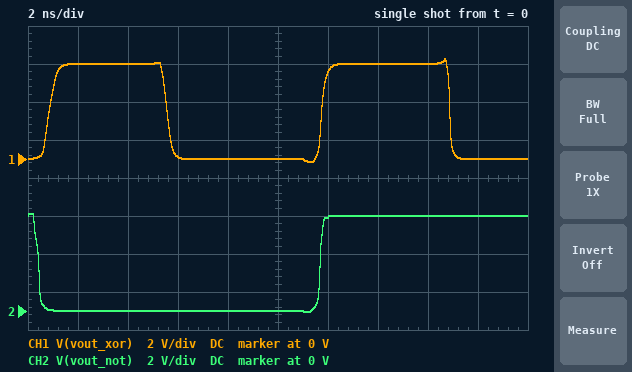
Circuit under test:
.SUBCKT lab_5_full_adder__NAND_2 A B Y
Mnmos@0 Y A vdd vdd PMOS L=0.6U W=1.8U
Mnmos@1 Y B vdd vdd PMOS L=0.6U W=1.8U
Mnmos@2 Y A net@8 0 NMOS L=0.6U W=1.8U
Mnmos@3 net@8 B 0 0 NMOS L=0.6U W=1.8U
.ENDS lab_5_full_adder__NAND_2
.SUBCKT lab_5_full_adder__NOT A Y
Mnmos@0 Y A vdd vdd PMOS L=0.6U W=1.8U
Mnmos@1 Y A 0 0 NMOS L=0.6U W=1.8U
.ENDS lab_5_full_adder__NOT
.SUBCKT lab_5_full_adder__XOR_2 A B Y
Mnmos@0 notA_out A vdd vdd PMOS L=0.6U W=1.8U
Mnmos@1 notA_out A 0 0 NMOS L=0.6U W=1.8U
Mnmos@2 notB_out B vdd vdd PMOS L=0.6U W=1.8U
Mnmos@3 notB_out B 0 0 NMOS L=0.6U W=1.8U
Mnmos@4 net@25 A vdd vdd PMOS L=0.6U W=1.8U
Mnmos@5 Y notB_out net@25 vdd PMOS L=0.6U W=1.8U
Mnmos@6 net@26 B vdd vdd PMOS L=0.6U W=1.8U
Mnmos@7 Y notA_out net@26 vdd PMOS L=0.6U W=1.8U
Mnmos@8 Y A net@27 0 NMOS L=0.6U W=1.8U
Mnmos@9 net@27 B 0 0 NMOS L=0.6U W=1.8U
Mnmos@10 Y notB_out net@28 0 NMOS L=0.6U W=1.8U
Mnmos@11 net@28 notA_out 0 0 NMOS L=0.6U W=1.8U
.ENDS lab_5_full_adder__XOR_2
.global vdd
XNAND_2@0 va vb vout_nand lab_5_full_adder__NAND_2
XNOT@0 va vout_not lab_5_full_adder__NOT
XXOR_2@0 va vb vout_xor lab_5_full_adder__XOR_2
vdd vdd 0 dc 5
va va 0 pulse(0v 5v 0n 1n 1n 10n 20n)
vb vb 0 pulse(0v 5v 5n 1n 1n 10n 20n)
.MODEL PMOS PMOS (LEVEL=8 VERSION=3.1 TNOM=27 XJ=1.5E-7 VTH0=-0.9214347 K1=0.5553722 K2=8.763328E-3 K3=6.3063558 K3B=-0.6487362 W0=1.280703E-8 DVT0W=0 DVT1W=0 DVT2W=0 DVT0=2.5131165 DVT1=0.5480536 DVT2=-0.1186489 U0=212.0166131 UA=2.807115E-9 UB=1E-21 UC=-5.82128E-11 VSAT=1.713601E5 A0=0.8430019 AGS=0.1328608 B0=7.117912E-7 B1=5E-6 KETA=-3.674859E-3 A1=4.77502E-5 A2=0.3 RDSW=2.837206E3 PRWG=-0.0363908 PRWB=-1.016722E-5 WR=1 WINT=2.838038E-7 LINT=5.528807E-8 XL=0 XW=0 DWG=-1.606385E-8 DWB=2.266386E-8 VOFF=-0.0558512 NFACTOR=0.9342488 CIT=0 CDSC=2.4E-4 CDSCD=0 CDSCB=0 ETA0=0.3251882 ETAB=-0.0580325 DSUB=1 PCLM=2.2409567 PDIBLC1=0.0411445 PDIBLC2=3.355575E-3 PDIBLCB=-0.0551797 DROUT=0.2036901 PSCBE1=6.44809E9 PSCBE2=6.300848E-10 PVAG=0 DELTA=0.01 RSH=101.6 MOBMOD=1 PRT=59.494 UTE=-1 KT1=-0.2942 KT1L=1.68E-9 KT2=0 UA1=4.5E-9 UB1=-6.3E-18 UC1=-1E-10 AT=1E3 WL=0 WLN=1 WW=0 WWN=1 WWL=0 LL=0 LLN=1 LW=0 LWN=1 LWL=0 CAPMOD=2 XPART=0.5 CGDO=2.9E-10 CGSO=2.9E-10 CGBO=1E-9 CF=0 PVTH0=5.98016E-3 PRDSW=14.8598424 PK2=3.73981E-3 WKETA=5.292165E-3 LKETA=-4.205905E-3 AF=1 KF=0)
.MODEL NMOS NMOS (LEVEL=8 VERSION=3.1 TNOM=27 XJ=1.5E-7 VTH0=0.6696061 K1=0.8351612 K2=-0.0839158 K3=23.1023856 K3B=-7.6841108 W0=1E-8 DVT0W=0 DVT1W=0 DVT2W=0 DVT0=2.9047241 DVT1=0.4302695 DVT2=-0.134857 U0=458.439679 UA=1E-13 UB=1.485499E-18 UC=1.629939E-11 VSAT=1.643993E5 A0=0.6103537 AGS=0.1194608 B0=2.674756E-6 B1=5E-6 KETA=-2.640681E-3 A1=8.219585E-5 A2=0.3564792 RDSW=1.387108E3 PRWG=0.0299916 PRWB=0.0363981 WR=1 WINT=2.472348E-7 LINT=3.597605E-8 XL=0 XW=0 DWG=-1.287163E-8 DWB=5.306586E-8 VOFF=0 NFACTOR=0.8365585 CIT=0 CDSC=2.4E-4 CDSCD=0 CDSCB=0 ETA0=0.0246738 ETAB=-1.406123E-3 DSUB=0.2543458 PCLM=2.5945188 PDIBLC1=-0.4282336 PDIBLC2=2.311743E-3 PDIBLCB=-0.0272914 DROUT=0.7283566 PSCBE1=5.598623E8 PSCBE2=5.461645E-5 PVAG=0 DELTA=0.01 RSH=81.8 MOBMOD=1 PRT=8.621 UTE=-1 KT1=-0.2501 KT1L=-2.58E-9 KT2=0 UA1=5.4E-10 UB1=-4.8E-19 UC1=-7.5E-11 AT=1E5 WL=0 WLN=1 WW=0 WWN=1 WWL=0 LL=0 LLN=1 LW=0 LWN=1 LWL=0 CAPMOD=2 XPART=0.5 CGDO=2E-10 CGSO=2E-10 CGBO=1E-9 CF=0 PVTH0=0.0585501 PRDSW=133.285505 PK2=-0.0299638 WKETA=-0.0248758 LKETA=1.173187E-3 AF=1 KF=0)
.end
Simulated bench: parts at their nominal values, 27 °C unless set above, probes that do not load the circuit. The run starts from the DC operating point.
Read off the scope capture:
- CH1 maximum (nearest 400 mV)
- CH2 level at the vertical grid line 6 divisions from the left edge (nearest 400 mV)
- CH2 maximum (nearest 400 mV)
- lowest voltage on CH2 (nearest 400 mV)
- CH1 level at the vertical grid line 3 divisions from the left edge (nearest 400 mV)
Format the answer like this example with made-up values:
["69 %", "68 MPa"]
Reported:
["5.2 V", "4.8 V", "5.2 V", "0 V", "0 V"]
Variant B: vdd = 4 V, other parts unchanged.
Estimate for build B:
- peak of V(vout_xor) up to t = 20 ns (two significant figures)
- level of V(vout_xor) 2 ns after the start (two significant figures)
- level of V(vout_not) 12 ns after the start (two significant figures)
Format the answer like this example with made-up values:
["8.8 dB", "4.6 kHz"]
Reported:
["4.4 V", "4.0 V", "3.9 V"]
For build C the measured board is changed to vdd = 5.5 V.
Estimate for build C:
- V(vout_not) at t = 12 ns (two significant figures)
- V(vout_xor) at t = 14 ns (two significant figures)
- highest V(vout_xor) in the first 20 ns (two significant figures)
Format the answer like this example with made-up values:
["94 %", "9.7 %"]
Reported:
["5.4 V", "5.5 V", "5.7 V"]
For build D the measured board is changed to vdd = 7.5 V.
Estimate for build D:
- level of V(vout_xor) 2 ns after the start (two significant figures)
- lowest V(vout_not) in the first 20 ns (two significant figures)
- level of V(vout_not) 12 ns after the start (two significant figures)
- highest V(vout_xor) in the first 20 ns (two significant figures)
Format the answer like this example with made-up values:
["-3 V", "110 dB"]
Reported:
["7.5 V", "300 mV", "7.4 V", "7.6 V"]
